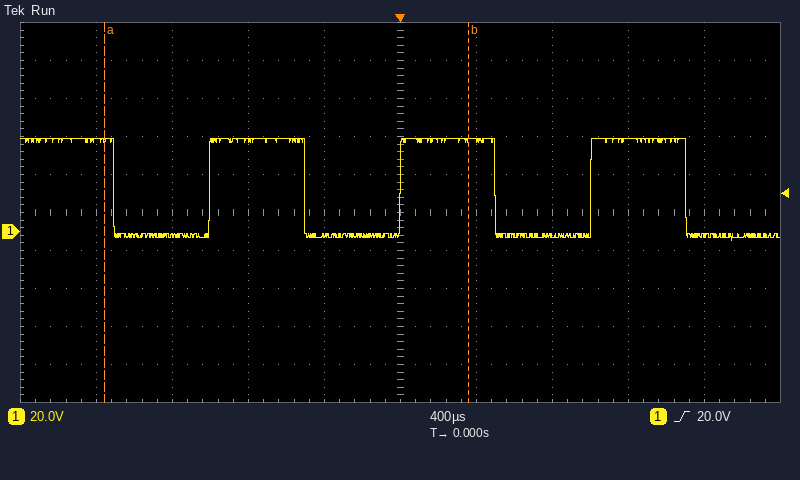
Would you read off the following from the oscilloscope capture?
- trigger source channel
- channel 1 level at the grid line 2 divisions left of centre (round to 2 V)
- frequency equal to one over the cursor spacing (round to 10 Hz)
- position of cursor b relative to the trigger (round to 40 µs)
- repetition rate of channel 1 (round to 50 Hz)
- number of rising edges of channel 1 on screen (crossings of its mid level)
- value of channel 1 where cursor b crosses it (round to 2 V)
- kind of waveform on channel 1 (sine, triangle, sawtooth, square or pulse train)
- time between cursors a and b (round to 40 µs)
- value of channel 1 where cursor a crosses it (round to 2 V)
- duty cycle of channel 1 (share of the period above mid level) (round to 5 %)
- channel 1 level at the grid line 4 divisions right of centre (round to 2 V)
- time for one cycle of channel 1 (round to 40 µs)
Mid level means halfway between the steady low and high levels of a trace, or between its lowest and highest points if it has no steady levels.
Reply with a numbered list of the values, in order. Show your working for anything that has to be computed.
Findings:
1. channel 1
2. 48 V
3. 1 / 1.92 ms ≈ 520 Hz
4. +360 µs
5. 1 / 1.00 ms ≈ 1.00 kHz
6. 3
7. 48 V
8. square
9. 1.92 ms
10. 48 V
11. 50 %
12. -2 V
13. 1.00 ms
